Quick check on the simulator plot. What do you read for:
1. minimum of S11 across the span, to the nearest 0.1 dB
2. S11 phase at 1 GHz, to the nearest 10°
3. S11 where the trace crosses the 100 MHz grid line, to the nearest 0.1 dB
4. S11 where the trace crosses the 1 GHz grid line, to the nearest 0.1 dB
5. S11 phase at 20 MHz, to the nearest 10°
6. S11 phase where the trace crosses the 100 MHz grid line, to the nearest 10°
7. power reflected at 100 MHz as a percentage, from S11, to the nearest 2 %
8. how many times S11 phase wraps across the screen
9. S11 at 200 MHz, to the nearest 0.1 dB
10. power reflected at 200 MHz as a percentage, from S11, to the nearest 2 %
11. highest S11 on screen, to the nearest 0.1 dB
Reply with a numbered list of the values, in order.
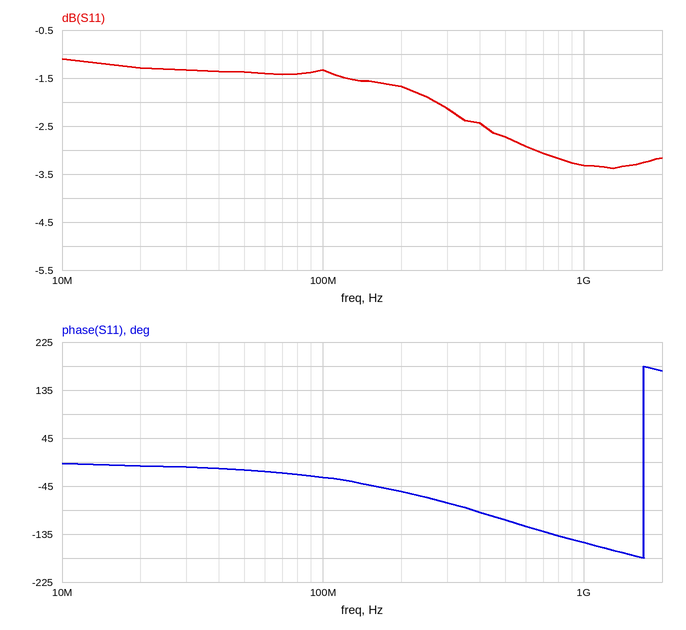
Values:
1. -3.4 dB
2. -150°
3. -1.3 dB
4. -3.3 dB
5. -10°
6. -30°
7. 74 %
8. 1
9. -1.7 dB
10. 68 %
11. -1.1 dB
